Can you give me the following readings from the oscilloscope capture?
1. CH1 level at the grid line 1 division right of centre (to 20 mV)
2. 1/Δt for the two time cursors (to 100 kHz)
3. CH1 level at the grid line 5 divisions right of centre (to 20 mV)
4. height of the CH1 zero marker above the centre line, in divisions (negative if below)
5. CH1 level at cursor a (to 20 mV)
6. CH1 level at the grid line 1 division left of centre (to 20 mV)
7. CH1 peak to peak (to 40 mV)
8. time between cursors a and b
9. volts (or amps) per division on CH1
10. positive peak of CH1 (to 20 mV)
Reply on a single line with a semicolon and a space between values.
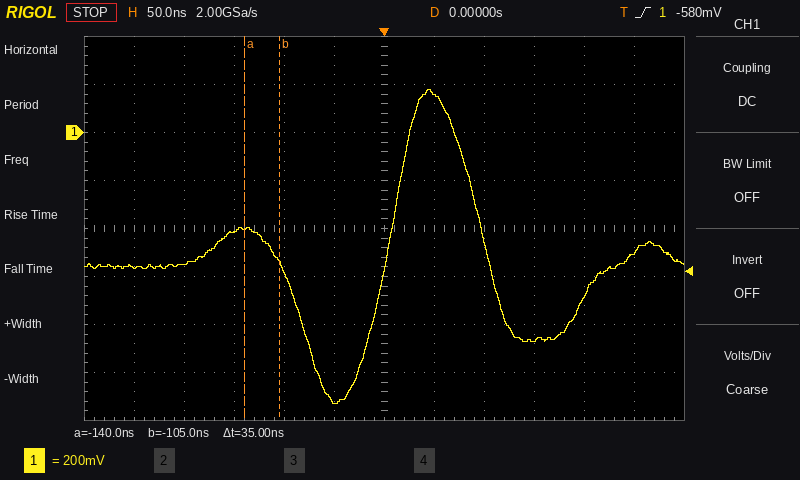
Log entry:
160 mV; 28.6 MHz; -500 mV; +2.0 div; -400 mV; -1.12 V; 1.32 V; 35 ns; 200 mV; 180 mV
